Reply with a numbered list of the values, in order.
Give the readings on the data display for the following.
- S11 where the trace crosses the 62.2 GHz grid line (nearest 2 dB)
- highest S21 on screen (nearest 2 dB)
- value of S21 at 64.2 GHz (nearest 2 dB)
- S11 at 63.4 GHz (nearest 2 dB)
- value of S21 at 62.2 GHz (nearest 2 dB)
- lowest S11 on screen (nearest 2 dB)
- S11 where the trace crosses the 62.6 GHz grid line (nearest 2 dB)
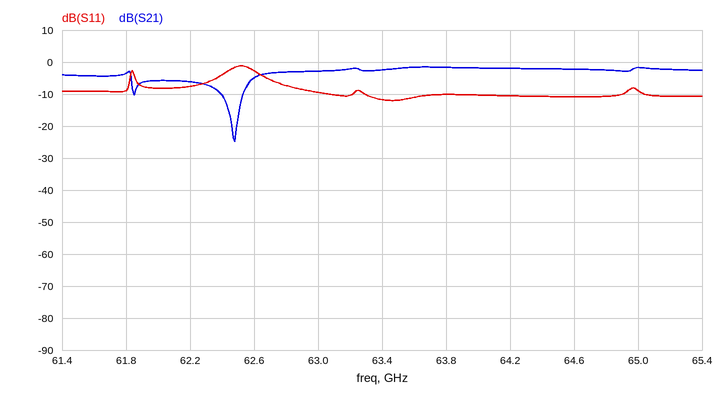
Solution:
1. -8 dB
2. -2 dB
3. -2 dB
4. -12 dB
5. -6 dB
6. -12 dB
7. -2 dB
